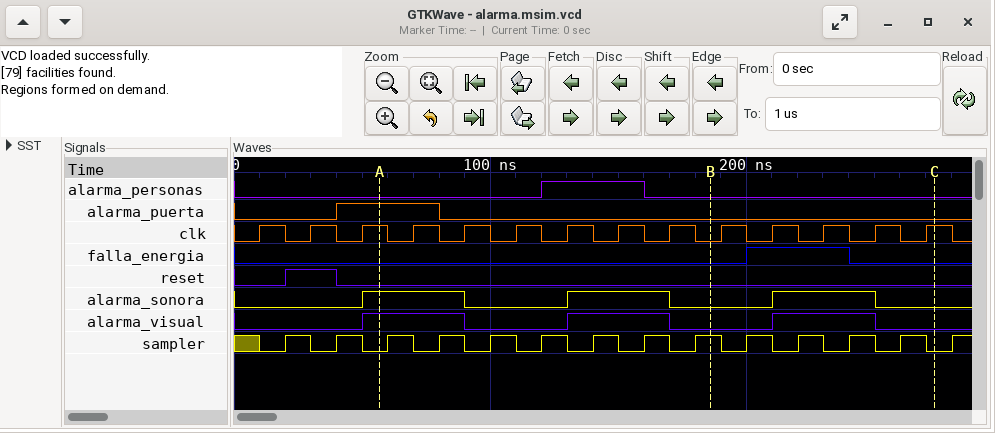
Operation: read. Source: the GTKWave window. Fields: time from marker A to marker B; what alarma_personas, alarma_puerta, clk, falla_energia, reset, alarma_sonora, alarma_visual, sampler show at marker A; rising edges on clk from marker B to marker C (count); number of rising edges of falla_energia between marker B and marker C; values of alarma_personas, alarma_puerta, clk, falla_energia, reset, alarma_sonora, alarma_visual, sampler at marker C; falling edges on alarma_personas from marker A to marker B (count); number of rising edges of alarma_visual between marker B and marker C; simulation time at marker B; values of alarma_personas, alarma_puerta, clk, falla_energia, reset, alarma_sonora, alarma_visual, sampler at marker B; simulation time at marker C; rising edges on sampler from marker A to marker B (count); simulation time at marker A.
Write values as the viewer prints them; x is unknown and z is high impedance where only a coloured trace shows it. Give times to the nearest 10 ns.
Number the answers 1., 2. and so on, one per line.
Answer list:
1. 130 ns
2. alarma_personas=0, alarma_puerta=1, clk=1, falla_energia=0, reset=0, alarma_sonora=1, alarma_visual=1, sampler=0
3. 5
4. 1
5. alarma_personas=0, alarma_puerta=0, clk=1, falla_energia=0, reset=0, alarma_sonora=0, alarma_visual=0, sampler=0
6. 1
7. 1
8. 190 ns
9. alarma_personas=0, alarma_puerta=0, clk=0, falla_energia=0, reset=0, alarma_sonora=0, alarma_visual=0, sampler=1
10. 270 ns
11. 7
12. 60 ns
